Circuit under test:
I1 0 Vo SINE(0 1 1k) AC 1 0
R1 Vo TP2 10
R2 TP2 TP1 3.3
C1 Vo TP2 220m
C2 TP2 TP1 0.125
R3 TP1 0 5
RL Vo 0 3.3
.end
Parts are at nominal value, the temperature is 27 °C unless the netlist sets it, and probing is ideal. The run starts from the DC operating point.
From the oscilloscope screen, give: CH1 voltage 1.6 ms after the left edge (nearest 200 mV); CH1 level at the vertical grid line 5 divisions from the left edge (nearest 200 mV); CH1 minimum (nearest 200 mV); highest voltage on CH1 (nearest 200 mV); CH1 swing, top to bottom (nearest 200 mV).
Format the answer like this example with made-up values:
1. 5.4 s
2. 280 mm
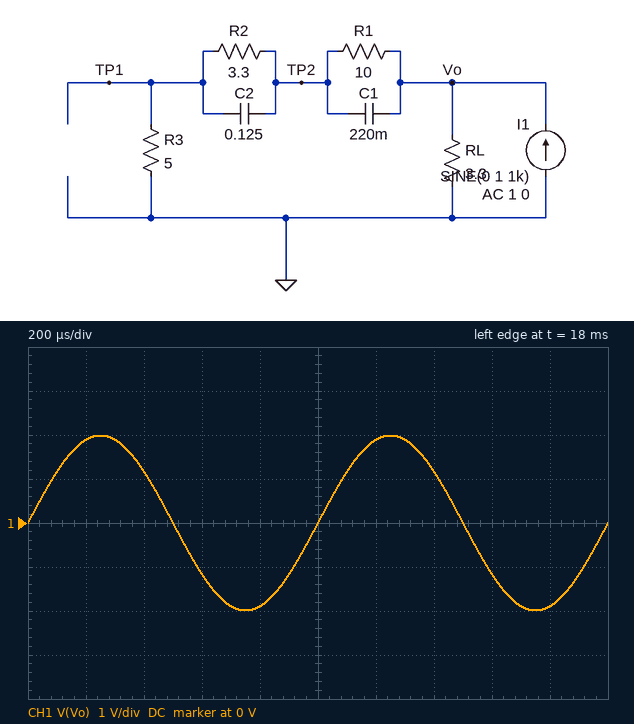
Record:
1. -1.2 V
2. 0 V
3. -2.0 V
4. 2.0 V
5. 4.0 V
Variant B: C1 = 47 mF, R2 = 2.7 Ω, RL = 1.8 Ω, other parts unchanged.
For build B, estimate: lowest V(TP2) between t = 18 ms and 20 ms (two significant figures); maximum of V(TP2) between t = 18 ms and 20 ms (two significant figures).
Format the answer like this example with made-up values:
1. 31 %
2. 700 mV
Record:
1. -1.3 V
2. 1.3 V
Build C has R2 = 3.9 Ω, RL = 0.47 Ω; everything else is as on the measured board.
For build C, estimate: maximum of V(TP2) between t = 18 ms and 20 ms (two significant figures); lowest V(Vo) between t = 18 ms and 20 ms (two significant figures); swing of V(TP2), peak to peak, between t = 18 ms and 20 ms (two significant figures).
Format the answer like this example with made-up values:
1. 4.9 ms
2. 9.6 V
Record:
1. 430 mV
2. -430 mV
3. 860 mV
